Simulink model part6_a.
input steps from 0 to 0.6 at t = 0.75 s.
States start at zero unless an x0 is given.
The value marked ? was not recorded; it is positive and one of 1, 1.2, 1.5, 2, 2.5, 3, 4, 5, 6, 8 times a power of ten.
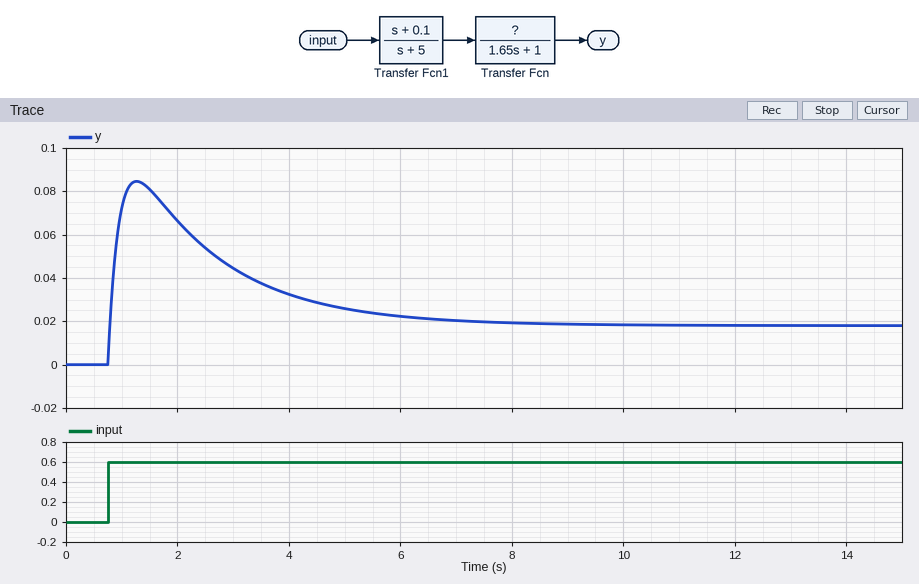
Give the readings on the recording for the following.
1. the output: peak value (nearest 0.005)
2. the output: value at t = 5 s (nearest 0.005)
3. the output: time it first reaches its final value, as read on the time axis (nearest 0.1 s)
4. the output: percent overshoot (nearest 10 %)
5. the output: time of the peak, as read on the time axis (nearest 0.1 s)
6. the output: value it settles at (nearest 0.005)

0.085
0.025
0.8 s
370 %
1.3 s
0.020
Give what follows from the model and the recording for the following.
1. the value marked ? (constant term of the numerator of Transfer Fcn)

1.5
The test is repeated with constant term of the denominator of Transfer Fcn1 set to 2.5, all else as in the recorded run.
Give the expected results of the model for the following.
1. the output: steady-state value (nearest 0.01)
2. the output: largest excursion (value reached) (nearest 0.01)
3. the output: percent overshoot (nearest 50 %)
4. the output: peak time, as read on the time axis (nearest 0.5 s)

0.04
0.15
300 %
1.5 s
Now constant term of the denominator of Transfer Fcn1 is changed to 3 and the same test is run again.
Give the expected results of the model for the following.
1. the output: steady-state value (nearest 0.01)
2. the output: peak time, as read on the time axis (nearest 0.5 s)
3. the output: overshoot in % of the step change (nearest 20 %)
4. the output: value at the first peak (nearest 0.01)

0.03
1.5 s
320 %
0.13
